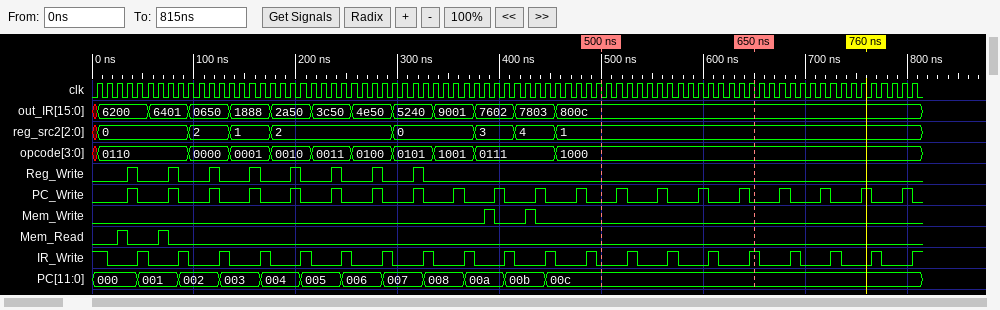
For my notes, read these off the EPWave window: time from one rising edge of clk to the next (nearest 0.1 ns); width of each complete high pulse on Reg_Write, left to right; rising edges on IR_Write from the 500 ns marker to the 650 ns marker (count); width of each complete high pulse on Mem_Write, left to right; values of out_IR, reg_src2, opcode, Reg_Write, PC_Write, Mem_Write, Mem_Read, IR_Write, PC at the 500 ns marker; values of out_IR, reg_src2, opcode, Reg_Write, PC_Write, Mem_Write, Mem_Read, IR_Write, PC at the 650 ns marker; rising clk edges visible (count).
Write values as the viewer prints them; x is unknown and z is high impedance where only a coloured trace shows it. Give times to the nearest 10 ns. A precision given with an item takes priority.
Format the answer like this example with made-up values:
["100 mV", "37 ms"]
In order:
["10 ns", "10 ns, 10 ns, 10 ns, 10 ns, 10 ns, 10 ns, 10 ns, 10 ns", "4", "10 ns, 10 ns", "out_IR=800c, reg_src2=1, opcode=1000, Reg_Write=0, PC_Write=0, Mem_Write=0, Mem_Read=0, IR_Write=0, PC=00c", "out_IR=800c, reg_src2=1, opcode=1000, Reg_Write=0, PC_Write=0, Mem_Write=0, Mem_Read=0, IR_Write=1, PC=00c", "81"]
